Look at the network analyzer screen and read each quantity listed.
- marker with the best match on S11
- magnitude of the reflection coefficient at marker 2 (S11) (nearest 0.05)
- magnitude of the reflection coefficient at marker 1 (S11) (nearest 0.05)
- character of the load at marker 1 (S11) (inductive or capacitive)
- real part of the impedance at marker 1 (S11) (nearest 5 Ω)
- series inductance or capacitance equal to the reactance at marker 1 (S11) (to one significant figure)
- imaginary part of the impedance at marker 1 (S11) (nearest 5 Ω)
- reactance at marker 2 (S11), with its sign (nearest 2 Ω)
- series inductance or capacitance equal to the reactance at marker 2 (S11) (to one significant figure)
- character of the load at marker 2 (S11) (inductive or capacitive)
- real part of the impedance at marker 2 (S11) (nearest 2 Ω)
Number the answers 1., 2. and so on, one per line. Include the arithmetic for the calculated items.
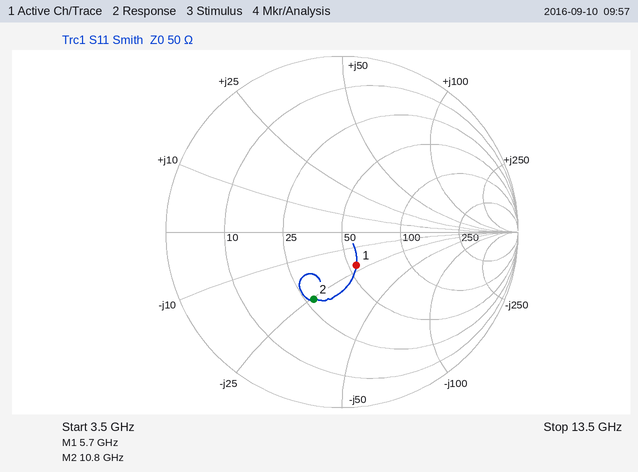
1. marker 1
2. 0.40
3. 0.20
4. capacitive
5. 55 Ω
6. C = 1/(2π × 5.7 GHz × 20 Ω) ≈ 1 pF
7. -20 Ω
8. -26 Ω
9. C = 1/(2π × 10.8 GHz × 26 Ω) ≈ 567 fF, so 600 fF to one significant figure
10. capacitive
11. 28 Ω
